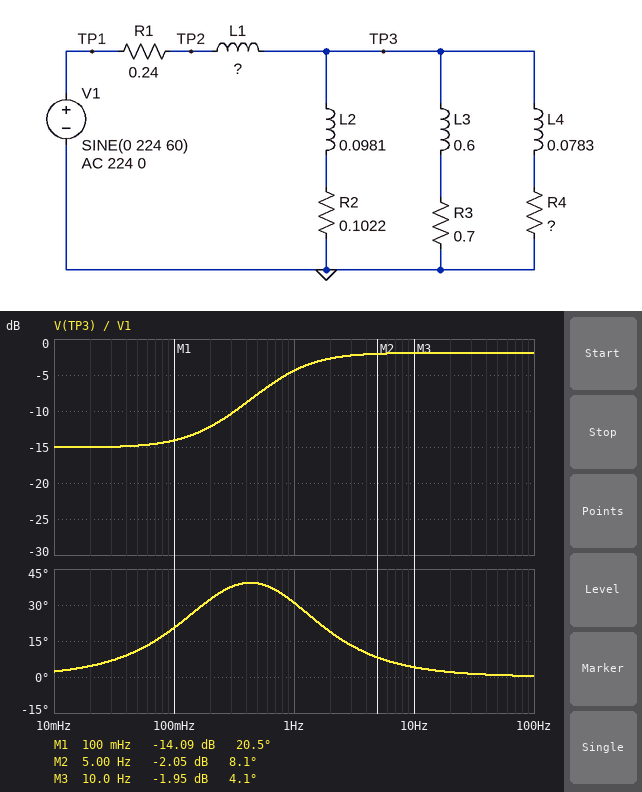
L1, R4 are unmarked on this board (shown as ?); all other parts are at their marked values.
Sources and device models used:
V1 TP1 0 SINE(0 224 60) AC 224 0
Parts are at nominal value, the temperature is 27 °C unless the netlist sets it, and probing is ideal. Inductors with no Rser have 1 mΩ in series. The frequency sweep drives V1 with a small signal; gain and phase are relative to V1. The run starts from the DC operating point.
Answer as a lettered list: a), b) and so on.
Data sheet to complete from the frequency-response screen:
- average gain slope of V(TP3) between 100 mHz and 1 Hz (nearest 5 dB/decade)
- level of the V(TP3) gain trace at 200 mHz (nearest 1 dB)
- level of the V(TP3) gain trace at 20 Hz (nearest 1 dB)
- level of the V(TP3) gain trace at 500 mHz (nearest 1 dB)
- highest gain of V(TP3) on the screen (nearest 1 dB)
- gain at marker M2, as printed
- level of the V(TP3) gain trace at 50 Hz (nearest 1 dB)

a) 10 dB/decade
b) -12 dB
c) -2 dB
d) -8 dB
e) -2 dB
f) -2.05 dB
g) -2 dB
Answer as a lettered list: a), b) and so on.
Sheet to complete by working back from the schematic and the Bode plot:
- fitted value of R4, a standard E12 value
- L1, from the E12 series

a) 0.12 Ω
b) 10 mH
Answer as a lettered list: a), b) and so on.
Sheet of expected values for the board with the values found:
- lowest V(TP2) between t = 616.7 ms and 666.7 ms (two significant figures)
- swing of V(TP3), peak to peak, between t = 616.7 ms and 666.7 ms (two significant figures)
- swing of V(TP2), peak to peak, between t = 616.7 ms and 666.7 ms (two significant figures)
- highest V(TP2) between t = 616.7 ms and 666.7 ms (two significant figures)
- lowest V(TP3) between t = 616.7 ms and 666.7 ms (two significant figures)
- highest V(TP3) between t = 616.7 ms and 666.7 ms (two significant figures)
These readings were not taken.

a) -220 V
b) 360 V
c) 450 V
d) 220 V
e) -180 V
f) 180 V
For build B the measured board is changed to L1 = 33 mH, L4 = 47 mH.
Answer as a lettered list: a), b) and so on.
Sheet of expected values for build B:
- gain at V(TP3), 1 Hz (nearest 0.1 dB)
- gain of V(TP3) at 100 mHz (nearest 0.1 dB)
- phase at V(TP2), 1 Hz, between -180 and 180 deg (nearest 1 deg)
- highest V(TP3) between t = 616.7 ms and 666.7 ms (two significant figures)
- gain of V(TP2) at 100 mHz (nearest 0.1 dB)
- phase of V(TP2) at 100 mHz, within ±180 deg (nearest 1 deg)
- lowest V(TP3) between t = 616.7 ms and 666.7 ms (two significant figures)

a) -7.9 dB
b) -14.3 dB
c) 28 deg
d) 110 V
e) -12.7 dB
f) 30 deg
g) -110 V
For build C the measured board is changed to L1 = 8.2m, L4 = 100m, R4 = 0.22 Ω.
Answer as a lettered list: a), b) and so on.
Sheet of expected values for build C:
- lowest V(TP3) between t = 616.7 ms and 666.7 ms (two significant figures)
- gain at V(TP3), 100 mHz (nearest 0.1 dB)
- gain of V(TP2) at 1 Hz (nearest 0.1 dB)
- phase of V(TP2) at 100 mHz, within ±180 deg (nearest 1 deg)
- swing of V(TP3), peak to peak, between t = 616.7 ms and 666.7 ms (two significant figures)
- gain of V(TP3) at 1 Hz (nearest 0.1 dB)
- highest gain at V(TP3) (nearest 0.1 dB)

a) -190 V
b) -12.6 dB
c) -2.5 dB
d) 22 deg
e) 380 V
f) -3.8 dB
g) -1.4 dB
